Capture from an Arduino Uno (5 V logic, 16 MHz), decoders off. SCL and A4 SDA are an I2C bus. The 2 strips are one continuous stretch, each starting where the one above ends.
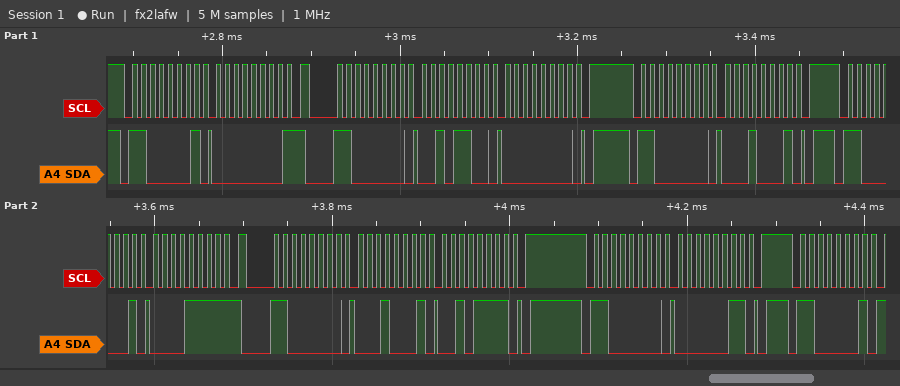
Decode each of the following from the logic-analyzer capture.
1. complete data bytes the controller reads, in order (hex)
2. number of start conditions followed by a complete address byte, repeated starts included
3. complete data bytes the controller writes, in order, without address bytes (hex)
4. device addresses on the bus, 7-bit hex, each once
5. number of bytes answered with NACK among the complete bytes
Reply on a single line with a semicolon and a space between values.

00 0F; 7; 2C 00 11 11 2F 03; 0x60; 2
